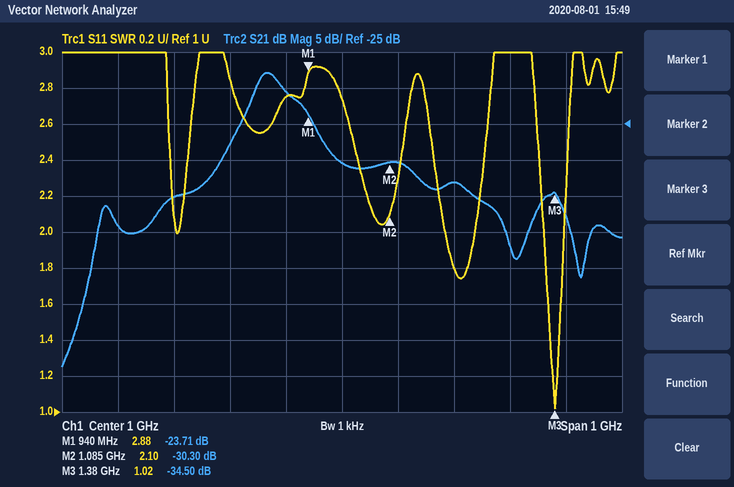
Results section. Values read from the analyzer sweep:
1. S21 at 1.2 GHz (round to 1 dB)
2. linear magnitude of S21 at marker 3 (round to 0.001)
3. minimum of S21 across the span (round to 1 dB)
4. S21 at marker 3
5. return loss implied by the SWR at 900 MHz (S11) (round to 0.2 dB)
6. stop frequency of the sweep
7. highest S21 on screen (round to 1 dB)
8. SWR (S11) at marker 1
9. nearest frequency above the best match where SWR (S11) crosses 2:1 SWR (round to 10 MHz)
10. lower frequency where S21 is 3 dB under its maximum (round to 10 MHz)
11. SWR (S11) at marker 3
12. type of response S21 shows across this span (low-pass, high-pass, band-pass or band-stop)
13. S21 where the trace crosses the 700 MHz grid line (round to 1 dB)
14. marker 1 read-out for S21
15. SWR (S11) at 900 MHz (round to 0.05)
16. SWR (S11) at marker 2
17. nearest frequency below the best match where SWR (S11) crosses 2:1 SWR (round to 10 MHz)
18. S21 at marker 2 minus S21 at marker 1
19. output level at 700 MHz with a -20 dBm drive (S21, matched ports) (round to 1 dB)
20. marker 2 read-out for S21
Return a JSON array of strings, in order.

["-33 dB", "0.019", "-59 dB", "-34.50 dB", "6.6 dB", "1.5 GHz", "-18 dB", "2.88", "1.40 GHz", "840 MHz", "1.02", "band-pass", "-35 dB", "-23.71 dB", "2.75", "2.10", "1.36 GHz", "-6.59 dB", "-55 dBm", "-30.30 dB"]
